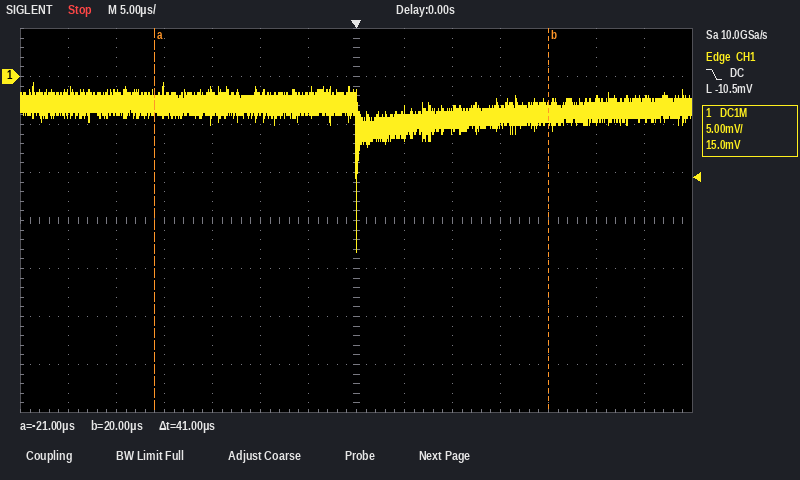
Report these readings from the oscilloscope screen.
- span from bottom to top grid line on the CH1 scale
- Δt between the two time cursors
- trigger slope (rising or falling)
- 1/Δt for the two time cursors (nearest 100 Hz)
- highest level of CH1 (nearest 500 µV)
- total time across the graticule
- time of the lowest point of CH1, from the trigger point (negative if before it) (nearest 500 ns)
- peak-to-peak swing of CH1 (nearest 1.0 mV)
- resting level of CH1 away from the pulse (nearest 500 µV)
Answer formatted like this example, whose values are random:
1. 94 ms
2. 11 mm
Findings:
1. 40 mV
2. 41 µs
3. falling
4. 24.4 kHz
5. -500 µV
6. 70 µs
7. 0.0 µs
8. 18.0 mV
9. -3.0 mV
